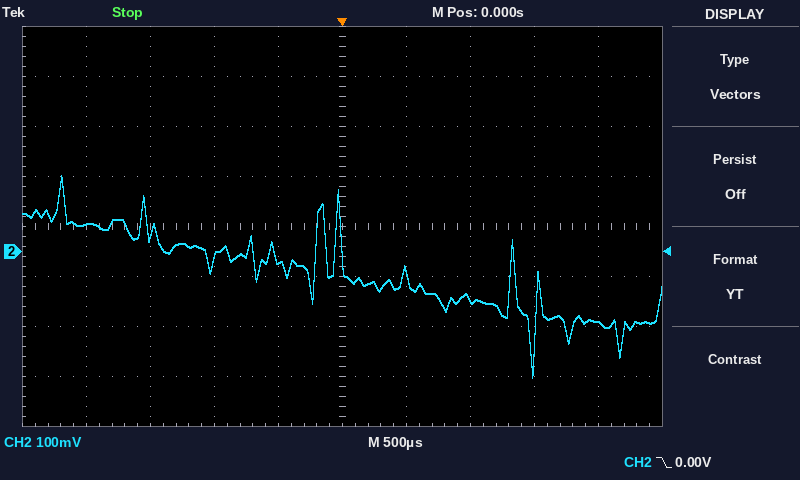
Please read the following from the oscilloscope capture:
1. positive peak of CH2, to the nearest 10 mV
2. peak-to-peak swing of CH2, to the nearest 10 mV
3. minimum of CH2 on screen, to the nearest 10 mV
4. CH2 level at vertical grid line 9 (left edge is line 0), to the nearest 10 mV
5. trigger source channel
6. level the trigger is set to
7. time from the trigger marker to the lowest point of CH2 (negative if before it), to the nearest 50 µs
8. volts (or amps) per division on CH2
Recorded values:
150 mV
400 mV
-250 mV
-140 mV
CH2
0.00 V
+1.50 ms
100 mV
